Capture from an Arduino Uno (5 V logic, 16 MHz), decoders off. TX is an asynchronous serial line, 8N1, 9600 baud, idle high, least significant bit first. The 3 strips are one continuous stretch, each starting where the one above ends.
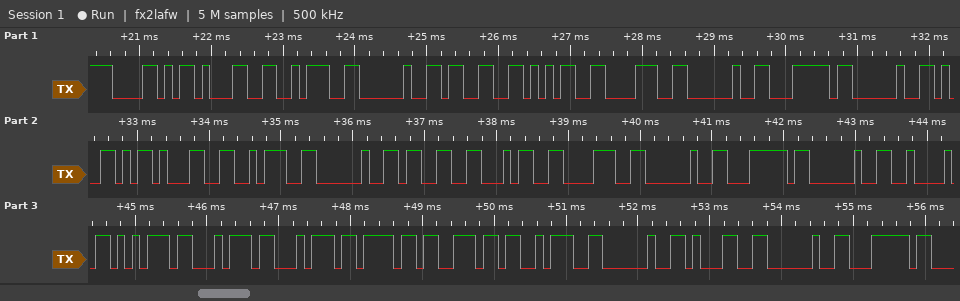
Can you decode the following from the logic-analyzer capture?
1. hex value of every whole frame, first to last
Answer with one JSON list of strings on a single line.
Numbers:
["58 31 3A 20 33 35 38 20 7C 20 59 31 3A 20 33 34 38 20 7C 20 42 75 74 74 6F 6E 3A 20 31 20 7C"]
